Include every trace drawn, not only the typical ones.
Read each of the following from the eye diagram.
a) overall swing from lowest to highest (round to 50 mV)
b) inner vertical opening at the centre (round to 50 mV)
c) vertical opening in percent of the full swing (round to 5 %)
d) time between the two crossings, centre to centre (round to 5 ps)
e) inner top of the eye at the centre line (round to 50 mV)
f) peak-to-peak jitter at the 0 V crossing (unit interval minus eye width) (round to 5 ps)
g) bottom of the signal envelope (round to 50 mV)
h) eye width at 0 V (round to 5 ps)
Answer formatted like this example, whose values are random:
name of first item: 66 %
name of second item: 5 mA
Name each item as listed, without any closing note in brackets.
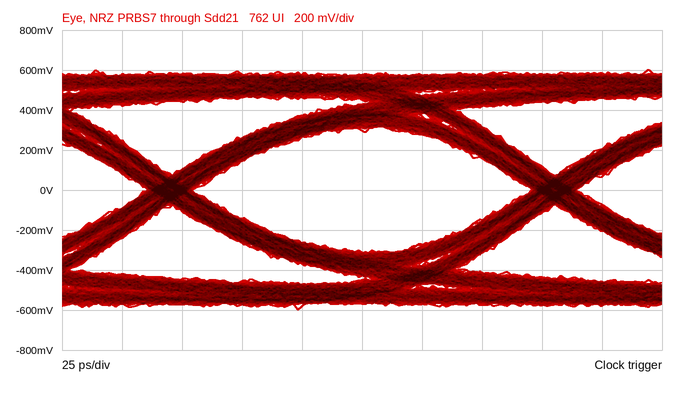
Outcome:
overall swing from lowest to highest: 1.20 V
inner vertical opening at the centre: 600 mV
vertical opening in percent of the full swing: 50 %
time between the two crossings, centre to centre: 160 ps
inner top of the eye at the centre line: 300 mV
peak-to-peak jitter at the 0 V crossing (unit interval minus eye width): 20 ps
bottom of the signal envelope: -600 mV
eye width at 0 V: 140 ps
